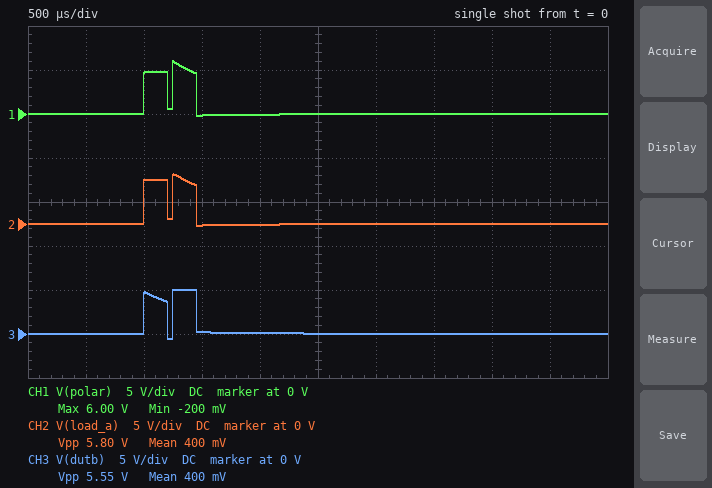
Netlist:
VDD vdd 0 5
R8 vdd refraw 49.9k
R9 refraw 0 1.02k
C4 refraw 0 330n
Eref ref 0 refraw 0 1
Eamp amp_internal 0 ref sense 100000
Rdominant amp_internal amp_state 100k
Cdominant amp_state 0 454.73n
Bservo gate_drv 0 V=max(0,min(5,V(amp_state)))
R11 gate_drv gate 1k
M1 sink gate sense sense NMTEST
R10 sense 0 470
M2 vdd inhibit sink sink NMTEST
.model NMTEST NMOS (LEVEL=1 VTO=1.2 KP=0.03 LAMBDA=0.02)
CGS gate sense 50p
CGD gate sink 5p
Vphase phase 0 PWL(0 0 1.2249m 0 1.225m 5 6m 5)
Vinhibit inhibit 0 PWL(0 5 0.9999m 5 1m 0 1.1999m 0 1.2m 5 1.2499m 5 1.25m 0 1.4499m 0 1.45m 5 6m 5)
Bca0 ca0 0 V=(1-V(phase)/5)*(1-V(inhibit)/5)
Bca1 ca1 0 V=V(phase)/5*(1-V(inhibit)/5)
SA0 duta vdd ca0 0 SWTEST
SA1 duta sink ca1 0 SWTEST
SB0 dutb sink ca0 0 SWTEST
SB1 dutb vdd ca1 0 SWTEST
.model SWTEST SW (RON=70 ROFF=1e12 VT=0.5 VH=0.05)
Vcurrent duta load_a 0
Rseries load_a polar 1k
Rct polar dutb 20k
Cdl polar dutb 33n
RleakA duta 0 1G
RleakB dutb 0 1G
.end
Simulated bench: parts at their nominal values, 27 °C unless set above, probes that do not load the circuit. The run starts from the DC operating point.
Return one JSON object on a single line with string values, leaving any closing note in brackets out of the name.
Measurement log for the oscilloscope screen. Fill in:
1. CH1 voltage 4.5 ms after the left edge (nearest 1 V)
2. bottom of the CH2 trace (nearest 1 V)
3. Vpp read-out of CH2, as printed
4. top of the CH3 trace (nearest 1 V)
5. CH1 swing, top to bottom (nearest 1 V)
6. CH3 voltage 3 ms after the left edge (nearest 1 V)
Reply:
{"CH1 voltage 4.5 ms after the left edge": "0 V", "bottom of the CH2 trace": "0 V", "Vpp read-out of CH2, as printed": "5.80 V", "top of the CH3 trace": "5 V", "CH1 swing, top to bottom": "6 V", "CH3 voltage 3 ms after the left edge": "0 V"}
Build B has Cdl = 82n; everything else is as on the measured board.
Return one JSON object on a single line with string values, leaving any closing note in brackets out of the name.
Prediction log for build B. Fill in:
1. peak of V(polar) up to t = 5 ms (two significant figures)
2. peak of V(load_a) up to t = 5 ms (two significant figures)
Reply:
{"peak of V(polar) up to t = 5 ms": "5.5 V", "peak of V(load_a) up to t = 5 ms": "5.3 V"}
